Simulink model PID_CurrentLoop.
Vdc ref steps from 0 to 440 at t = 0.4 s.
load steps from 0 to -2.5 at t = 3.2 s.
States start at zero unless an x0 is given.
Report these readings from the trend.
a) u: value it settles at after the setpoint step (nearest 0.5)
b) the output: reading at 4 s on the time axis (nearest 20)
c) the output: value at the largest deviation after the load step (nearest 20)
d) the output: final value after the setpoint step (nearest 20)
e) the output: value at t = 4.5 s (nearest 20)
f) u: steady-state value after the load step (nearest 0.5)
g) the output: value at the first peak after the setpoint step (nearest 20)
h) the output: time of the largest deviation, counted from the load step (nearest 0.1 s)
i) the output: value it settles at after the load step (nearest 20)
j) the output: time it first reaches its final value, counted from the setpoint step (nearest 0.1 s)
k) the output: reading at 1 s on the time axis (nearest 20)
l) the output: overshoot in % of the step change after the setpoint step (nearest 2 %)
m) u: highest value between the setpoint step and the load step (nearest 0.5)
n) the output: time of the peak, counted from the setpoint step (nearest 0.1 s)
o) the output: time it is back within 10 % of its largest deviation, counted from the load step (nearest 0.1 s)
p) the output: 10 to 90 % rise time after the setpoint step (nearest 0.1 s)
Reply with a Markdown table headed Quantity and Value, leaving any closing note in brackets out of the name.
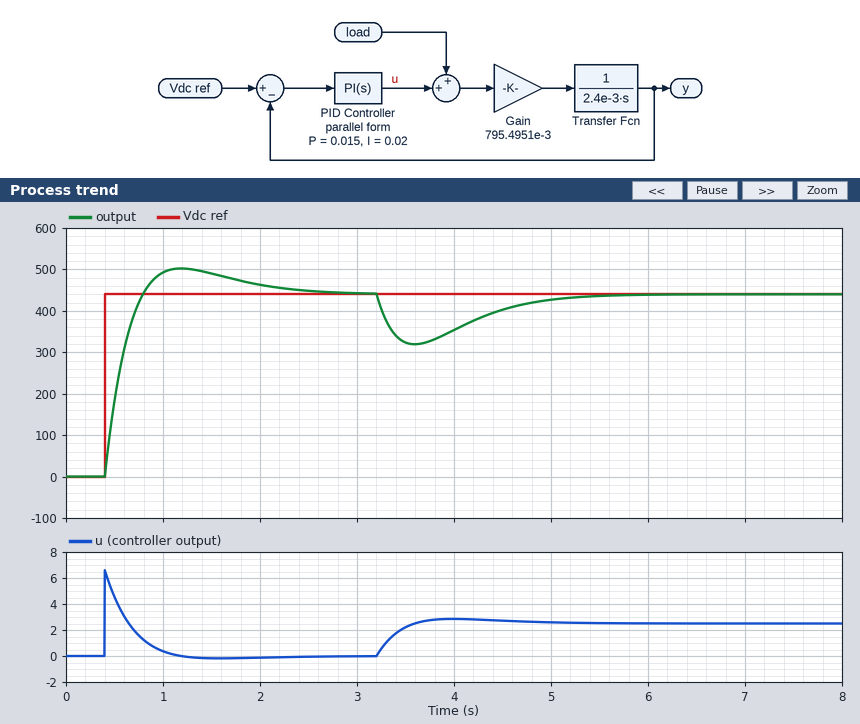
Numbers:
| Quantity | Value |
|---|---|
| u: value it settles at after the setpoint step | 0.0 |
| the output: reading at 4 s on the time axis | 360 |
| the output: value at the largest deviation after the load step | 320 |
| the output: final value after the setpoint step | 440 |
| the output: value at t = 4.5 s | 400 |
| u: steady-state value after the load step | 2.5 |
| the output: value at the first peak after the setpoint step | 500 |
| the output: time of the largest deviation, counted from the load step | 0.4 s |
| the output: value it settles at after the load step | 440 |
| the output: time it first reaches its final value, counted from the setpoint step | 0.4 s |
| the output: reading at 1 s on the time axis | 500 |
| the output: overshoot in % of the step change after the setpoint step | 14 % |
| u: highest value between the setpoint step and the load step | 6.5 |
| the output: time of the peak, counted from the setpoint step | 0.8 s |
| the output: time it is back within 10 % of its largest deviation, counted from the load step | 1.8 s |
| the output: 10 to 90 % rise time after the setpoint step | 0.3 s |
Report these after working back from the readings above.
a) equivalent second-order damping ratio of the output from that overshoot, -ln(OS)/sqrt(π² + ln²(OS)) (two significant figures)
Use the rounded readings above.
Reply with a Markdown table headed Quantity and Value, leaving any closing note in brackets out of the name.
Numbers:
| Quantity | Value |
|---|---|
| equivalent second-order damping ratio of the output from that overshoot, -ln(OS)/sqrt(π² + ln²(OS)) | 0.53 |
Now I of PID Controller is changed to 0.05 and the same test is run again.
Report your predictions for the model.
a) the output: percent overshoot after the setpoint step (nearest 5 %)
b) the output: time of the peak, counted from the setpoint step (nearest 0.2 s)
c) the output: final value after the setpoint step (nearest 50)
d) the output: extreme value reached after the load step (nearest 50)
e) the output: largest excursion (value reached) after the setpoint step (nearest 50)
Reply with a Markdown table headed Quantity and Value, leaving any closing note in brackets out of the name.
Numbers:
| Quantity | Value |
|---|---|
| the output: percent overshoot after the setpoint step | 25 % |
| the output: time of the peak, counted from the setpoint step | 0.6 s |
| the output: final value after the setpoint step | 450 |
| the output: extreme value reached after the load step | 350 |
| the output: largest excursion (value reached) after the setpoint step | 550 |
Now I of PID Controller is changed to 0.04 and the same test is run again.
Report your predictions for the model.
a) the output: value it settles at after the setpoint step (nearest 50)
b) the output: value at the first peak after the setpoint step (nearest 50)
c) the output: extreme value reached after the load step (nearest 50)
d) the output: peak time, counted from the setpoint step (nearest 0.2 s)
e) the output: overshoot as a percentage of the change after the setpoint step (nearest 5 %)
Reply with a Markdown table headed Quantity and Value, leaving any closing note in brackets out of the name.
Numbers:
| Quantity | Value |
|---|---|
| the output: value it settles at after the setpoint step | 450 |
| the output: value at the first peak after the setpoint step | 550 |
| the output: extreme value reached after the load step | 350 |
| the output: peak time, counted from the setpoint step | 0.6 s |
| the output: overshoot as a percentage of the change after the setpoint step | 20 % |
